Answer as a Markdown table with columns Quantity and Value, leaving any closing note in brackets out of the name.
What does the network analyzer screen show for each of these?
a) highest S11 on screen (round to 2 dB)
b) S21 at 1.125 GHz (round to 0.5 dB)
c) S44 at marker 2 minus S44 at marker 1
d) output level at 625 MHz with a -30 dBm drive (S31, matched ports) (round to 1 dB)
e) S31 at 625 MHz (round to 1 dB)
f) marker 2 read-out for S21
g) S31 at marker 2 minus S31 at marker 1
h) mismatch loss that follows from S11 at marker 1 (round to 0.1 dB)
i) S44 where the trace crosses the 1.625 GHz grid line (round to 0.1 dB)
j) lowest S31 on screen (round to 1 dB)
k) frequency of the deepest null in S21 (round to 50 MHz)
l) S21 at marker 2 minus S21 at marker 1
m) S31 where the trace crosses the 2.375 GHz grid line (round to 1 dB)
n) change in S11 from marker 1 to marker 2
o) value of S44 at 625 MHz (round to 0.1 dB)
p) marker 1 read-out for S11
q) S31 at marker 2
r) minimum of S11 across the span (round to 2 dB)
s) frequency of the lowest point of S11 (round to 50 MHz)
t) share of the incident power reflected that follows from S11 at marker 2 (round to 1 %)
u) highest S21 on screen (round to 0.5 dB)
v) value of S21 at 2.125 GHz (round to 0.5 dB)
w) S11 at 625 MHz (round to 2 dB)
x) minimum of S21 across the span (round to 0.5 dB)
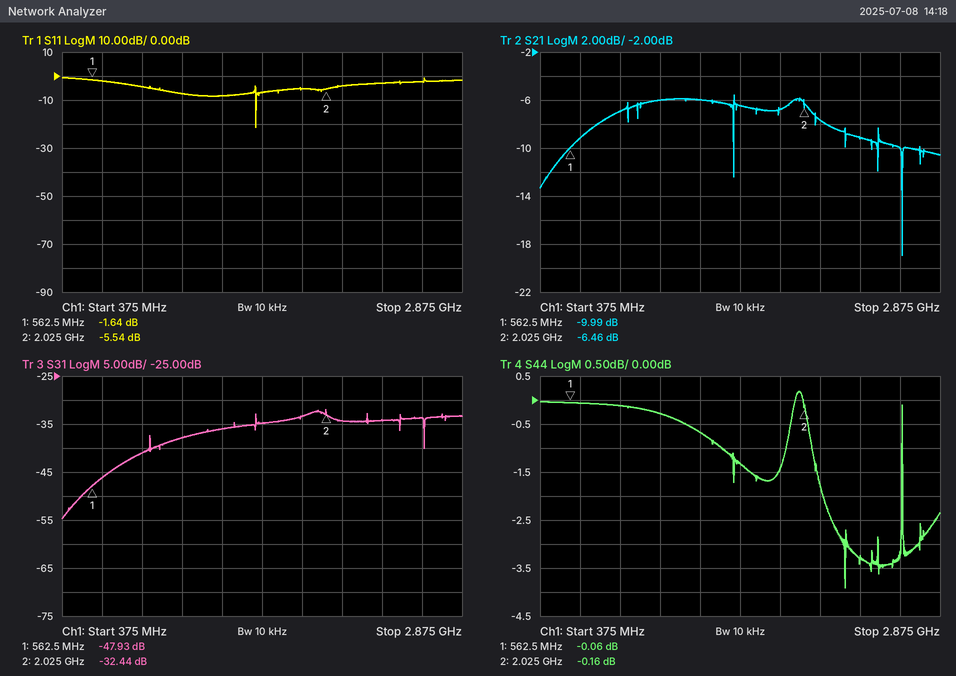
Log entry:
| Quantity | Value |
|---|---|
| highest S11 on screen | 0 dB |
| S21 at 1.125 GHz | -6.0 dB |
| S44 at marker 2 minus S44 at marker 1 | -0.10 dB |
| output level at 625 MHz with a -30 dBm drive (S31, matched ports) | -76 dBm |
| S31 at 625 MHz | -46 dB |
| marker 2 read-out for S21 | -6.46 dB |
| S31 at marker 2 minus S31 at marker 1 | 15.49 dB |
| mismatch loss that follows from S11 at marker 1 | 5.0 dB |
| S44 where the trace crosses the 1.625 GHz grid line | -1.3 dB |
| lowest S31 on screen | -55 dB |
| frequency of the deepest null in S21 | 2.65 GHz |
| S21 at marker 2 minus S21 at marker 1 | 3.53 dB |
| S31 where the trace crosses the 2.375 GHz grid line | -34 dB |
| change in S11 from marker 1 to marker 2 | -3.90 dB |
| value of S44 at 625 MHz | -0.1 dB |
| marker 1 read-out for S11 | -1.64 dB |
| S31 at marker 2 | -32.44 dB |
| minimum of S11 across the span | -22 dB |
| frequency of the lowest point of S11 | 1.60 GHz |
| share of the incident power reflected that follows from S11 at marker 2 | 28 % |
| highest S21 on screen | -5.5 dB |
| value of S21 at 2.125 GHz | -7.5 dB |
| S11 at 625 MHz | -2 dB |
| minimum of S21 across the span | -19.0 dB |
